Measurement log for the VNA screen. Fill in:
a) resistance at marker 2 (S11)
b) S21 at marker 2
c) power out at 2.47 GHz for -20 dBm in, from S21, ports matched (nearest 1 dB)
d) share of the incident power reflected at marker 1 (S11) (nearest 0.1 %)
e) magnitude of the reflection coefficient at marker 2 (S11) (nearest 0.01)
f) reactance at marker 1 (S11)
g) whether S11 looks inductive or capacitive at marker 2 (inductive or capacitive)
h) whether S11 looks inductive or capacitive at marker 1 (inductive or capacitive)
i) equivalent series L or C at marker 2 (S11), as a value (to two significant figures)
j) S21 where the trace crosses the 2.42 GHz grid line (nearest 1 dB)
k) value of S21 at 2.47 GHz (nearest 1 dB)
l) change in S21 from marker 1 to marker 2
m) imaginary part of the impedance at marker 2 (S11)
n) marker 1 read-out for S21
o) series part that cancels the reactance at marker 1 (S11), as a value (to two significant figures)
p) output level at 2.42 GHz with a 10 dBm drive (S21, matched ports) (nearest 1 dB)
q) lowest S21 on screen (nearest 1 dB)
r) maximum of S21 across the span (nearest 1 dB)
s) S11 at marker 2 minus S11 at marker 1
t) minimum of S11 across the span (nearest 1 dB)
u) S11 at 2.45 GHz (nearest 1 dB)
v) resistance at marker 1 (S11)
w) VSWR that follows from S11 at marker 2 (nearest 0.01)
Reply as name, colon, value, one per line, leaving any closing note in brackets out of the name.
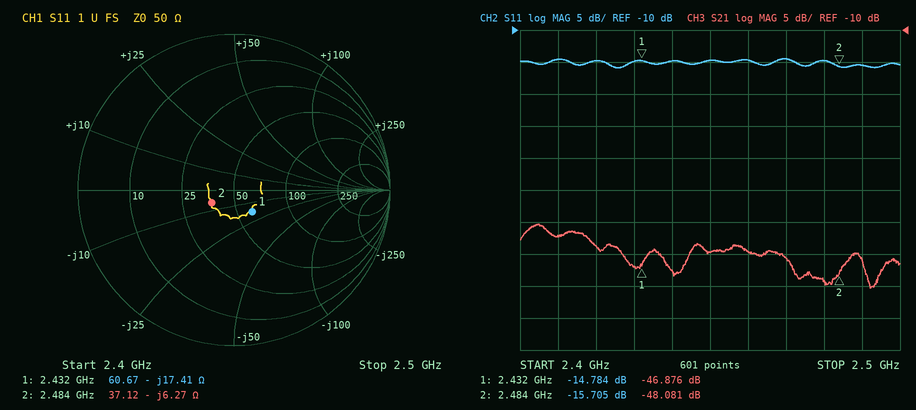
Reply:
resistance at marker 2: 37.12 Ω
S21 at marker 2: -48.081 dB
power out at 2.47 GHz for -20 dBm in, from S21, ports matched: -66 dBm
share of the incident power reflected at marker 1 (S11): 3.3 %
magnitude of the reflection coefficient at marker 2 (S11): 0.16
reactance at marker 1: -17.41 Ω
whether S11 looks inductive or capacitive at marker 2: capacitive
whether S11 looks inductive or capacitive at marker 1: capacitive
equivalent series L or C at marker 2 (S11), as a value: 10 pF
S21 where the trace crosses the 2.42 GHz grid line: -44 dB
value of S21 at 2.47 GHz: -46 dB
change in S21 from marker 1 to marker 2: -1.205 dB
imaginary part of the impedance at marker 2: -6.27 Ω
marker 1 read-out for S21: -46.876 dB
series part that cancels the reactance at marker 1 (S11), as a value: 1.1 nH
output level at 2.42 GHz with a 10 dBm drive (S21, matched ports): -34 dBm
lowest S21 on screen: -50 dB
maximum of S21 across the span: -40 dB
S11 at marker 2 minus S11 at marker 1: -0.921 dB
minimum of S11 across the span: -16 dB
S11 at 2.45 GHz: -15 dB
resistance at marker 1: 60.67 Ω
VSWR that follows from S11 at marker 2: 1.39
